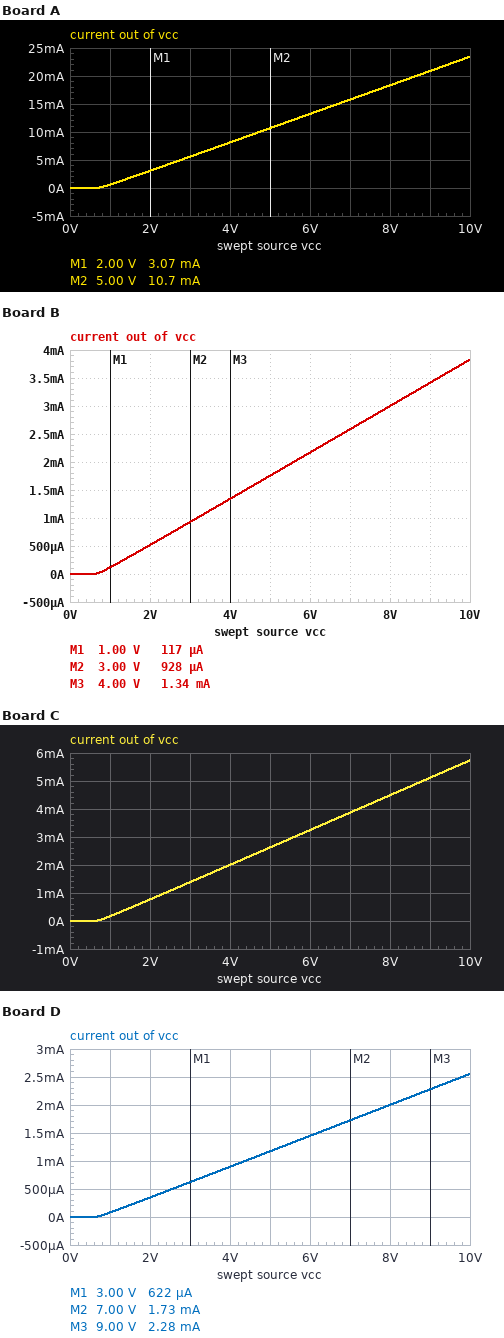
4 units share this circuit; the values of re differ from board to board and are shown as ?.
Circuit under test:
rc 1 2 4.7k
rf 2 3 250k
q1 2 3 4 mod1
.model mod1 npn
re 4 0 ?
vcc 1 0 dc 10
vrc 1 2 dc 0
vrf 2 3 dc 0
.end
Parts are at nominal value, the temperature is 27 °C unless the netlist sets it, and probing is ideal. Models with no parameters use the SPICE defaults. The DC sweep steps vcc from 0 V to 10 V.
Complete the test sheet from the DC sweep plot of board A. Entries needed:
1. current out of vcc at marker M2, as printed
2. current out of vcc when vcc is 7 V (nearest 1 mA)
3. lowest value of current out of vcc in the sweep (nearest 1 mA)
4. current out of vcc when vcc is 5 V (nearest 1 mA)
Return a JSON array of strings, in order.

["10.7 mA", "16 mA", "0 A", "11 mA"]
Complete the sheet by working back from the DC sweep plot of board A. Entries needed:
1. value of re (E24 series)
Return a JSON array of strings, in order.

["390 Ω"]
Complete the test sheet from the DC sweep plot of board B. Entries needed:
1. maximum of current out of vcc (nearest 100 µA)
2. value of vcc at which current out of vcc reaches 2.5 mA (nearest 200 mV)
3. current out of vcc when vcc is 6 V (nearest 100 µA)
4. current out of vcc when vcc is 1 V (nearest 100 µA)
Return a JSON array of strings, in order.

["3.8 mA", "6.8 V", "2.2 mA", "100 µA"]
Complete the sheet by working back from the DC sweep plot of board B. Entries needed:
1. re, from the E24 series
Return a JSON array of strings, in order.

["2.4 kΩ"]
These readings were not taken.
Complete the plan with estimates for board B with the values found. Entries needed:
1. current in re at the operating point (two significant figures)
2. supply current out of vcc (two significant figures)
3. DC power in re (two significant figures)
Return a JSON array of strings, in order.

["3.8 mA", "3.8 mA", "35 mW"]
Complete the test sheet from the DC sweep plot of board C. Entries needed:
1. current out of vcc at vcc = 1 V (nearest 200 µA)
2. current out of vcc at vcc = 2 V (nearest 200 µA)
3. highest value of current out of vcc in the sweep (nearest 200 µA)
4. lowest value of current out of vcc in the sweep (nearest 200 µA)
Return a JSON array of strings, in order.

["200 µA", "800 µA", "5.8 mA", "0 A"]
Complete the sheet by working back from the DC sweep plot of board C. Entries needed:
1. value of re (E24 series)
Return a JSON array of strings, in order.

["1.6 kΩ"]
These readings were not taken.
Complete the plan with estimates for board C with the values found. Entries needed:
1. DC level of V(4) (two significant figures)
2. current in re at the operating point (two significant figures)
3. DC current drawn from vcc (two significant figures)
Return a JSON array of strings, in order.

["9.2 V", "5.7 mA", "5.7 mA"]
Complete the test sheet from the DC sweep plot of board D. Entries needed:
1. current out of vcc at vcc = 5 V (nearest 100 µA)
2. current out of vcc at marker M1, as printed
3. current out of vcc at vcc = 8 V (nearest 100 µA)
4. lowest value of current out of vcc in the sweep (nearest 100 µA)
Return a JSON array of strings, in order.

["1.2 mA", "622 µA", "2.0 mA", "0 A"]
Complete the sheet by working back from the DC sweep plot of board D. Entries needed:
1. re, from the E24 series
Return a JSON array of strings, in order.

["3.6 kΩ"]
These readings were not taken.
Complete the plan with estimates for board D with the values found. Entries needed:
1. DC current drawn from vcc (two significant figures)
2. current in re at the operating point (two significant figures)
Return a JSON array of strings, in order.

["2.6 mA", "2.6 mA"]
